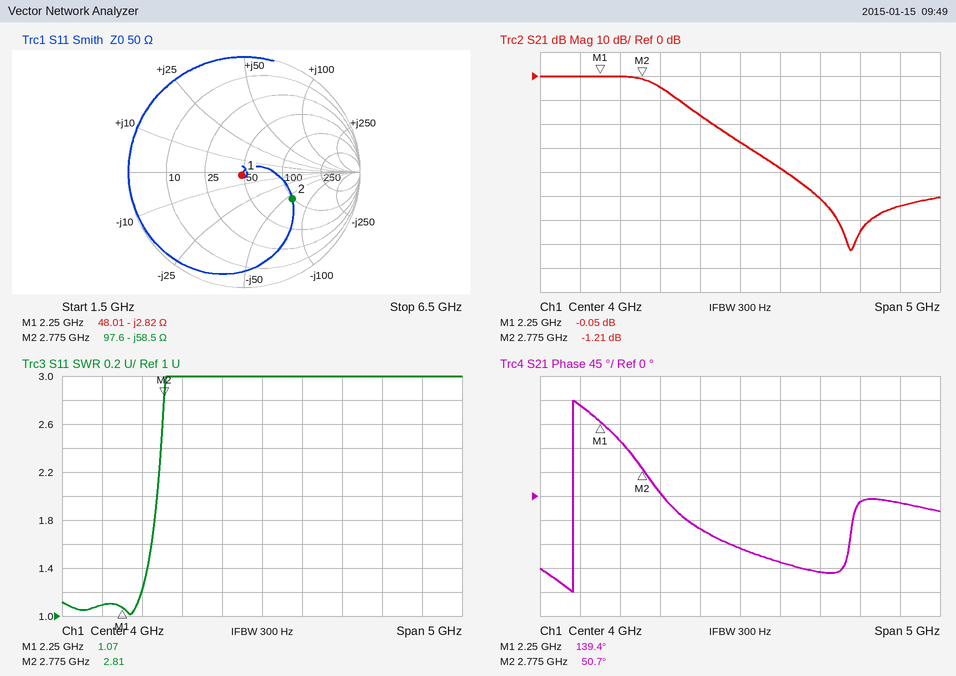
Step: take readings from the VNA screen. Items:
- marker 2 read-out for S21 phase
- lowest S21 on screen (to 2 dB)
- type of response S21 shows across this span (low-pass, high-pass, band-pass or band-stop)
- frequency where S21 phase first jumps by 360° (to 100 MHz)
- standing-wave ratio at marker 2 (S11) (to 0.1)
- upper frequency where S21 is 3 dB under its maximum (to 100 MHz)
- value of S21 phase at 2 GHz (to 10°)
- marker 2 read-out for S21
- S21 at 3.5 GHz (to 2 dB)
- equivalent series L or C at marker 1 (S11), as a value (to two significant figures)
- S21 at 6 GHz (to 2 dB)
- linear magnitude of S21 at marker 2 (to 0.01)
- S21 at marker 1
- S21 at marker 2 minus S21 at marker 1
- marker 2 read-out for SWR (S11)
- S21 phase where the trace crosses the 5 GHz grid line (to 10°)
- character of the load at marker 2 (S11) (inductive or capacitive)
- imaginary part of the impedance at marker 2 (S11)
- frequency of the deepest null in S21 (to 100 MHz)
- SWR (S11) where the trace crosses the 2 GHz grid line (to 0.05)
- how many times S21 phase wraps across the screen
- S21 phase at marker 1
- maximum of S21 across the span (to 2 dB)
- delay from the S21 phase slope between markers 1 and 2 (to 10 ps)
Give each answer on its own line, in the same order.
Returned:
50.7°
-72 dB
low-pass
1.9 GHz
2.8
2.9 GHz
170°
-1.21 dB
-16 dB
25 pF
-54 dB
0.87
-0.05 dB
-1.16 dB
2.81
-140°
capacitive
-58.5 Ω
5.4 GHz
1.10
1
139.4°
0 dB
470 ps
